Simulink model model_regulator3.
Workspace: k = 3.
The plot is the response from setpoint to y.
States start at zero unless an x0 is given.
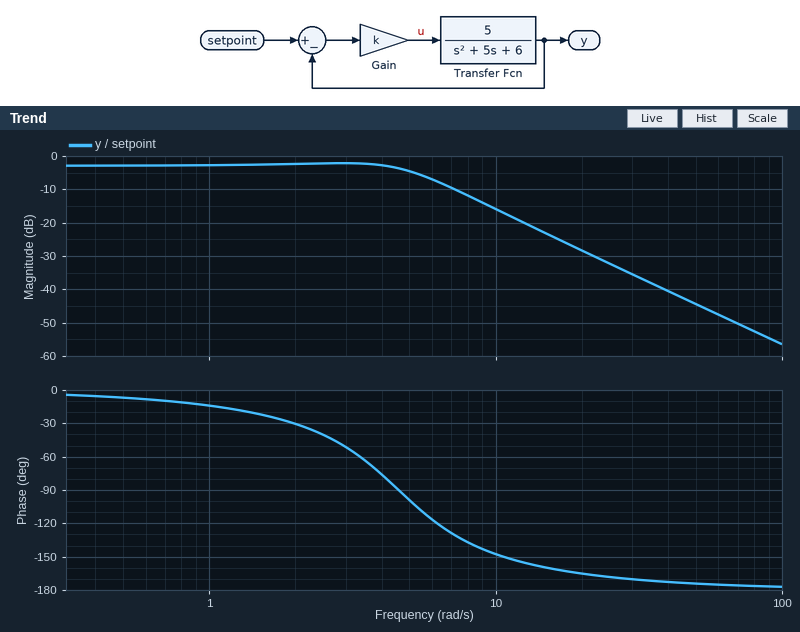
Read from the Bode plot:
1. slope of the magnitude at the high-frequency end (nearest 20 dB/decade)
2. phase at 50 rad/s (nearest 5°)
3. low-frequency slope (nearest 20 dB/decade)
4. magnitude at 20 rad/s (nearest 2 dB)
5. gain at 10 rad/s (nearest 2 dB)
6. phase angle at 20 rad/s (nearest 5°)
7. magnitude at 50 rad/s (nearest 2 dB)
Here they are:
-40 dB/decade
-175°
0 dB/decade
-28 dB
-16 dB
-165°
-44 dB
